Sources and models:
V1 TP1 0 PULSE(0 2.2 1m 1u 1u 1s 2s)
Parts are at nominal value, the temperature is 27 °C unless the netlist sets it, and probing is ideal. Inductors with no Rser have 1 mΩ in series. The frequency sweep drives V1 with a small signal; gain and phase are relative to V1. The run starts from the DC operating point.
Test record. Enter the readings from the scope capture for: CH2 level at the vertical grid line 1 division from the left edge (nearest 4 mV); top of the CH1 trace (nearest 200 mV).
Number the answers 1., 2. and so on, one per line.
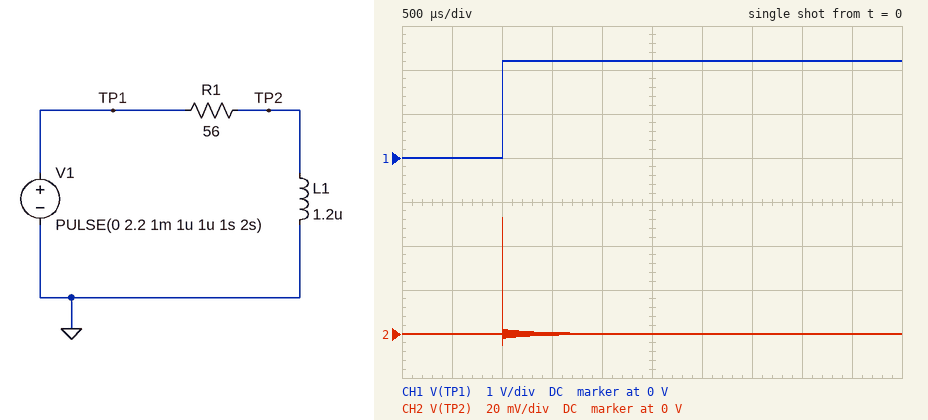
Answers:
1. 0 V
2. 2.2 V
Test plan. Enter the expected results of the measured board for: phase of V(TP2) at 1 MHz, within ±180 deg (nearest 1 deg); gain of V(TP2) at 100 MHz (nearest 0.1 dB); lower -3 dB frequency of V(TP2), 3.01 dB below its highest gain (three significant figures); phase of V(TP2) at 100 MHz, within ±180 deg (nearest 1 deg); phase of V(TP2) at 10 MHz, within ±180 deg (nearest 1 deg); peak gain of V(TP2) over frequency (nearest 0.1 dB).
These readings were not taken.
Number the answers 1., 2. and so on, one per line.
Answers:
1. 82 deg
2. 0 dB
3. 7.43 MHz
4. 4 deg
5. 37 deg
6. 0 dB
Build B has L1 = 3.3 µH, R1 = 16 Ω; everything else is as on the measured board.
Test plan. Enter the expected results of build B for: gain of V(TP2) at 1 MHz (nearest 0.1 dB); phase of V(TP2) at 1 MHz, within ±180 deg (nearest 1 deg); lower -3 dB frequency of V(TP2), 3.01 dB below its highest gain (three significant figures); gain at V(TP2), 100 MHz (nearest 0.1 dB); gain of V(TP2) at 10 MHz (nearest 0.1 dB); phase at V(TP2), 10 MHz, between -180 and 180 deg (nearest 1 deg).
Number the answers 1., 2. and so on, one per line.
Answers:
1. -2.0 dB
2. 38 deg
3. 772 kHz
4. 0 dB
5. 0 dB
6. 4 deg
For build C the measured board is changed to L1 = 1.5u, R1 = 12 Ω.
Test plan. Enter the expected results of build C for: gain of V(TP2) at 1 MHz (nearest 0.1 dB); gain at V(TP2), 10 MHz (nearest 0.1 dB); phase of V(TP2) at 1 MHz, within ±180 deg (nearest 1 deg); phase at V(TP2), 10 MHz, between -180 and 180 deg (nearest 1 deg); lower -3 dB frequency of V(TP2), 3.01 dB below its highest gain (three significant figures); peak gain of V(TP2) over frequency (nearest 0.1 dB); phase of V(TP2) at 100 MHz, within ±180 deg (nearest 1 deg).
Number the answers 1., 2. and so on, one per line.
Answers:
1. -4.2 dB
2. -0.1 dB
3. 52 deg
4. 7 deg
5. 1.27 MHz
6. 0 dB
7. 1 deg
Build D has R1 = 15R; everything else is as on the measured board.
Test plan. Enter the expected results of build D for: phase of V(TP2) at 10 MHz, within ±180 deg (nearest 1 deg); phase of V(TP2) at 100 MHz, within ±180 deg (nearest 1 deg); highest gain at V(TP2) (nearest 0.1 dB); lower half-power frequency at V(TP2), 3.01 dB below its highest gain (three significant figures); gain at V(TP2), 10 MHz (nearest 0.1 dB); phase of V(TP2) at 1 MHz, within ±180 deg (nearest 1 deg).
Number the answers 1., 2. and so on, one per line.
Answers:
1. 11 deg
2. 1 deg
3. 0 dB
4. 1.99 MHz
5. -0.2 dB
6. 63 deg
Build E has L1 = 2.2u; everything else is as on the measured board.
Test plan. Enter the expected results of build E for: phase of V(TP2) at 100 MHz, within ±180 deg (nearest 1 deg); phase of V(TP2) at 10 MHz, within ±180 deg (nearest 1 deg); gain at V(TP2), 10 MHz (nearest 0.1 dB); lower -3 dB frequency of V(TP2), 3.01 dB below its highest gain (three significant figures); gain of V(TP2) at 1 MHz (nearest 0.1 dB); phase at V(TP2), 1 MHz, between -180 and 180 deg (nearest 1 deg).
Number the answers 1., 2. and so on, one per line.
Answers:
1. 2 deg
2. 22 deg
3. -0.7 dB
4. 4.05 MHz
5. -12.4 dB
6. 76 deg
